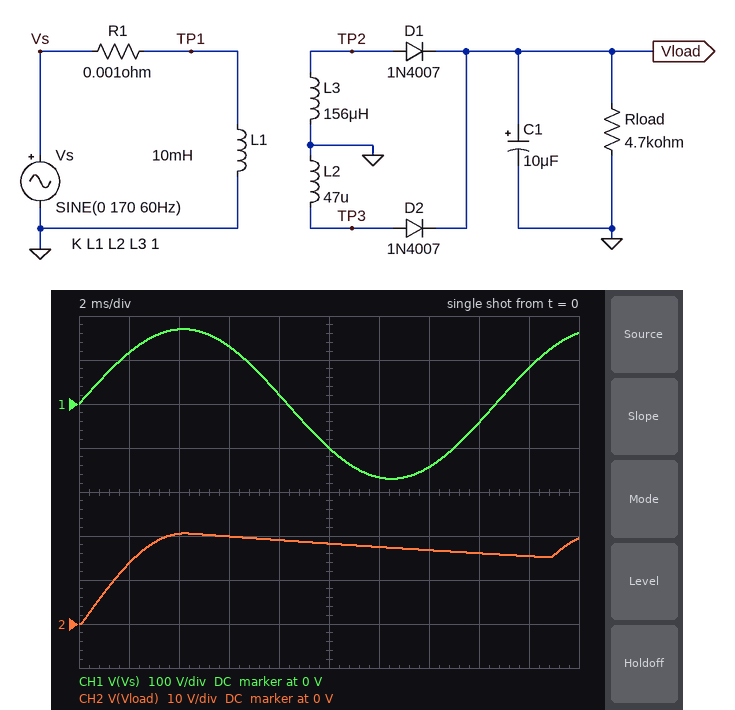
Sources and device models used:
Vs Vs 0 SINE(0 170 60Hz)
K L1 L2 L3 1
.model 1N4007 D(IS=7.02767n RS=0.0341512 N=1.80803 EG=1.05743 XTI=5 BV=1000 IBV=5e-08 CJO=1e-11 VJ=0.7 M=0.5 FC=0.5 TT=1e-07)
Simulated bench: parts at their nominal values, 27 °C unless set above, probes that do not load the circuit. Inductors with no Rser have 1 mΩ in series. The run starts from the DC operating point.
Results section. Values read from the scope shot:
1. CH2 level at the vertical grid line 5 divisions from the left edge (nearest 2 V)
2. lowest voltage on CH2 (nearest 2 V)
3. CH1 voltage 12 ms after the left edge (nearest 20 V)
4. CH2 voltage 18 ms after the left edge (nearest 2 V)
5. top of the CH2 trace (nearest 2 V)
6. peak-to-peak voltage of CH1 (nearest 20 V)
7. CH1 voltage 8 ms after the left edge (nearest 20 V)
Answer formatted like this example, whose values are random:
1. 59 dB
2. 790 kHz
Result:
1. 18 V
2. 0 V
3. -160 V
4. 16 V
5. 20 V
6. 340 V
7. 20 V
